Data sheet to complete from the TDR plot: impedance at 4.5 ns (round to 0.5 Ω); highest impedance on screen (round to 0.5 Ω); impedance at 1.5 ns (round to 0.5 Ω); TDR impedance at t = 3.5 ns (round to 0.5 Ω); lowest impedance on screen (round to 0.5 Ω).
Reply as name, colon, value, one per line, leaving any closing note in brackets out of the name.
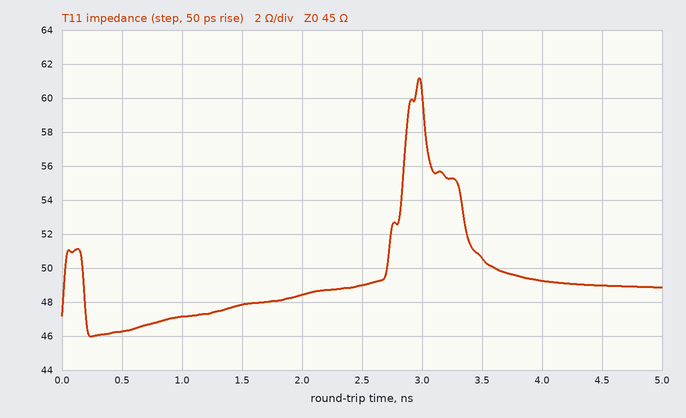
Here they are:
impedance at 4.5 ns: 49.0 Ω
highest impedance on screen: 61.0 Ω
impedance at 1.5 ns: 48.0 Ω
TDR impedance at t = 3.5 ns: 50.5 Ω
lowest impedance on screen: 46.0 Ω
